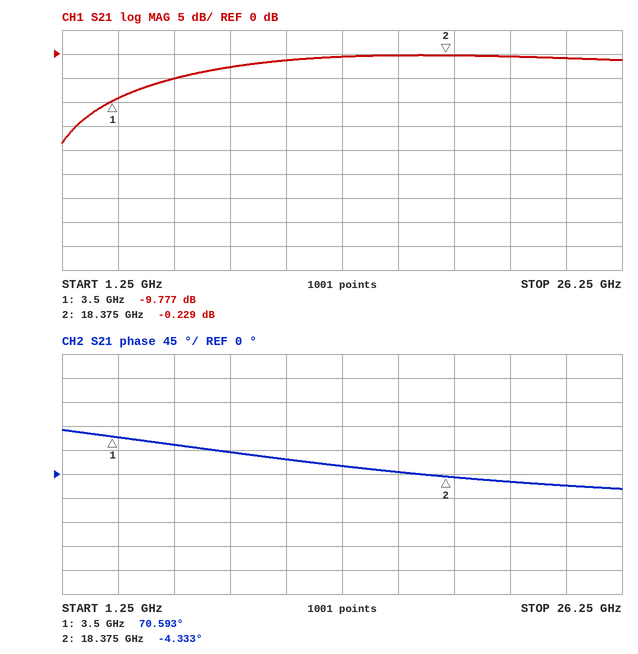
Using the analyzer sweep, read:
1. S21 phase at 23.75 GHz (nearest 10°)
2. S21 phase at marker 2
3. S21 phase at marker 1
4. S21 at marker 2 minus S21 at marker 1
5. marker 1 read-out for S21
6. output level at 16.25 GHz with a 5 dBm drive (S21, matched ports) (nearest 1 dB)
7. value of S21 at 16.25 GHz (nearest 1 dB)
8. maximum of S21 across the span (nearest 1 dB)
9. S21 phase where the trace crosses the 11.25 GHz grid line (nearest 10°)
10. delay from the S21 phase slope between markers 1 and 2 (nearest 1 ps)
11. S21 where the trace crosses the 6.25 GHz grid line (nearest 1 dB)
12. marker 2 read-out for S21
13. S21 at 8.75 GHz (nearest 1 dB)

-20°
-4.333°
70.593°
9.548 dB
-9.777 dB
5 dBm
0 dB
0 dB
30°
14 ps
-5 dB
-0.229 dB
-3 dB
